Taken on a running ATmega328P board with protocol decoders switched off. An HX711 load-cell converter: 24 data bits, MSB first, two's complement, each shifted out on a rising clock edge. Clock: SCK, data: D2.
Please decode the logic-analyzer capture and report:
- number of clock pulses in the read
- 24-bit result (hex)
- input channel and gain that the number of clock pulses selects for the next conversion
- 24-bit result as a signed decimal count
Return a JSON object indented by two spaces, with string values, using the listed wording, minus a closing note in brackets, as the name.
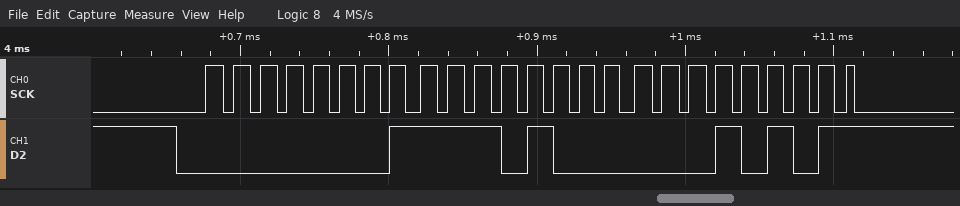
{
  "number of clock pulses in the read": "25",
  "24-bit result": "0x01E815",
  "input channel and gain that the number of clock pulses selects for the next conversion": "channel A, gain 128",
  "24-bit result as a signed decimal count": "124949"
}
